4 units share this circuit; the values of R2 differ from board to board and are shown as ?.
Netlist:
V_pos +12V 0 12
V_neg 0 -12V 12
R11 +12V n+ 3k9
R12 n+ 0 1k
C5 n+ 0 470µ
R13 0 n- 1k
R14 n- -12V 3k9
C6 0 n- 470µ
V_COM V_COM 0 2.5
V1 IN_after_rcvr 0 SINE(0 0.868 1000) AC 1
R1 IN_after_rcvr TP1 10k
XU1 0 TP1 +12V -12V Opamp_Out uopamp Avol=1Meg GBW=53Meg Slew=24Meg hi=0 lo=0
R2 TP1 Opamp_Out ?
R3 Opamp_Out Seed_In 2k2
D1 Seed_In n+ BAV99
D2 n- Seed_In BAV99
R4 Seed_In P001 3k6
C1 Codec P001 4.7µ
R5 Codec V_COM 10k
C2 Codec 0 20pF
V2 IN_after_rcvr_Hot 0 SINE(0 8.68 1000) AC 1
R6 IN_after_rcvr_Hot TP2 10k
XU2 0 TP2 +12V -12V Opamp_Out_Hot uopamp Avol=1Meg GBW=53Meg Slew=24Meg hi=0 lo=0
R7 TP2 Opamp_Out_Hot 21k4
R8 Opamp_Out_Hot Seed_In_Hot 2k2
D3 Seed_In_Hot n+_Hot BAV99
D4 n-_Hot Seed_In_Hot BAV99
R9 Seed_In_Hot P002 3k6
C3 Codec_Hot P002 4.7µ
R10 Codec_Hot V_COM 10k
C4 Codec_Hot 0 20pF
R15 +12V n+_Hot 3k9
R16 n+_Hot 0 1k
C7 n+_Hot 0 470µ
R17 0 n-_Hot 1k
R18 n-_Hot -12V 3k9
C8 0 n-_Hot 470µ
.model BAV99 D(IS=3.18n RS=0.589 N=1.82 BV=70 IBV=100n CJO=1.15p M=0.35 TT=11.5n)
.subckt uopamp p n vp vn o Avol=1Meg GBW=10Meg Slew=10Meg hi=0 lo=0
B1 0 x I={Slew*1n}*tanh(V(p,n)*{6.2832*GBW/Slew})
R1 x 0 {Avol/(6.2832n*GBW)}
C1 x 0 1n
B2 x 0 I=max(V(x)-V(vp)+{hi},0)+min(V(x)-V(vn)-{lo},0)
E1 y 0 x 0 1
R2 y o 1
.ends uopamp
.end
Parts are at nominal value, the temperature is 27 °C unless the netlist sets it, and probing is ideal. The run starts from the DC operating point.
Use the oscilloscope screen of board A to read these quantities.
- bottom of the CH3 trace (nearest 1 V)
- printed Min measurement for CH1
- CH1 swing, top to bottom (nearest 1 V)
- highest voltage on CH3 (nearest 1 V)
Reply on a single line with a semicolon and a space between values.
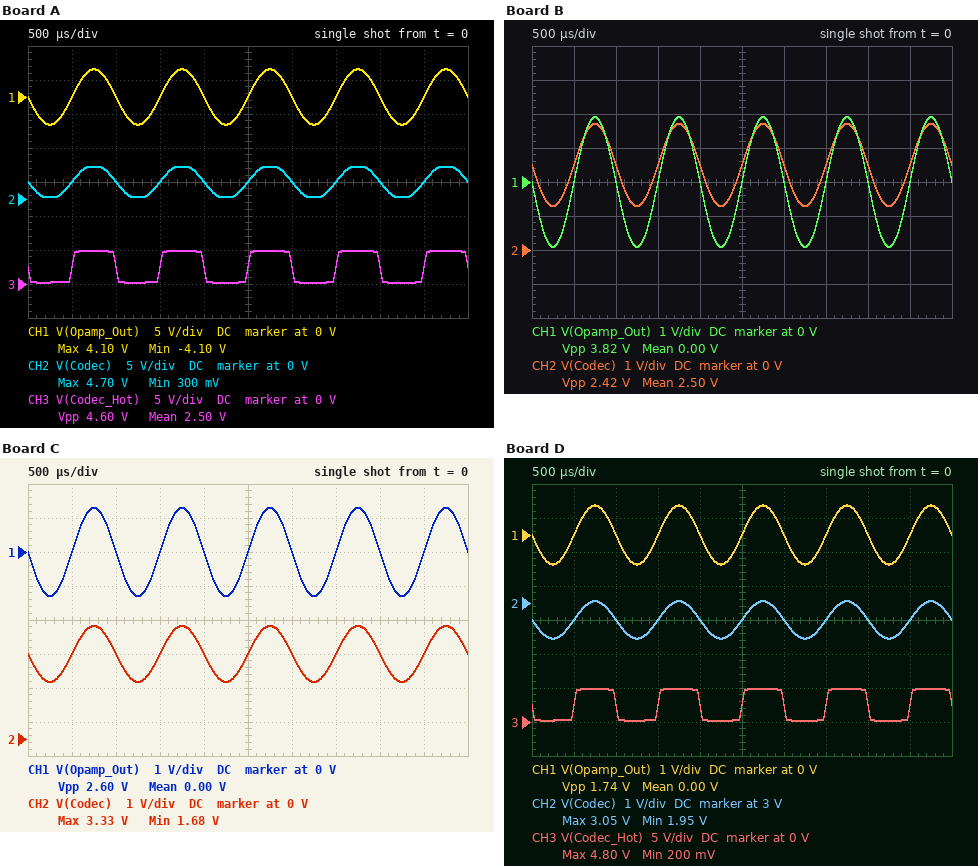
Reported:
0 V; -4.10 V; 8 V; 5 V
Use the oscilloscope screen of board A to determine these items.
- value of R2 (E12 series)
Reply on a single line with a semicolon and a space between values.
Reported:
47 kΩ
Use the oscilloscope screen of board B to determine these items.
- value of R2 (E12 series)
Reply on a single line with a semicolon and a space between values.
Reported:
22 kΩ
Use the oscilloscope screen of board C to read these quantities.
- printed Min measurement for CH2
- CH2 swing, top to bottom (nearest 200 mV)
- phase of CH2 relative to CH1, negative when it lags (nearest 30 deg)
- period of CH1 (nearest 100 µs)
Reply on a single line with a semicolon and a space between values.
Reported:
1.68 V; 1.6 V; 0 deg; 1.0 ms
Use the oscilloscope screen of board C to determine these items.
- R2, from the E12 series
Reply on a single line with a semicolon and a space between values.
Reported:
15 kΩ
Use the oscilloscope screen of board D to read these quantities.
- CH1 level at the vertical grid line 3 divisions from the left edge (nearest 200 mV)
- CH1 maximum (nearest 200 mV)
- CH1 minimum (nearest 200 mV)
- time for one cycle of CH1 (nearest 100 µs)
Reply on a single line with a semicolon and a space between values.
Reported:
0 V; 800 mV; -800 mV; 1.0 ms
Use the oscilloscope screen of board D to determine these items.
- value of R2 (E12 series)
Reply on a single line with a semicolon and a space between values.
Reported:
10 kΩ
